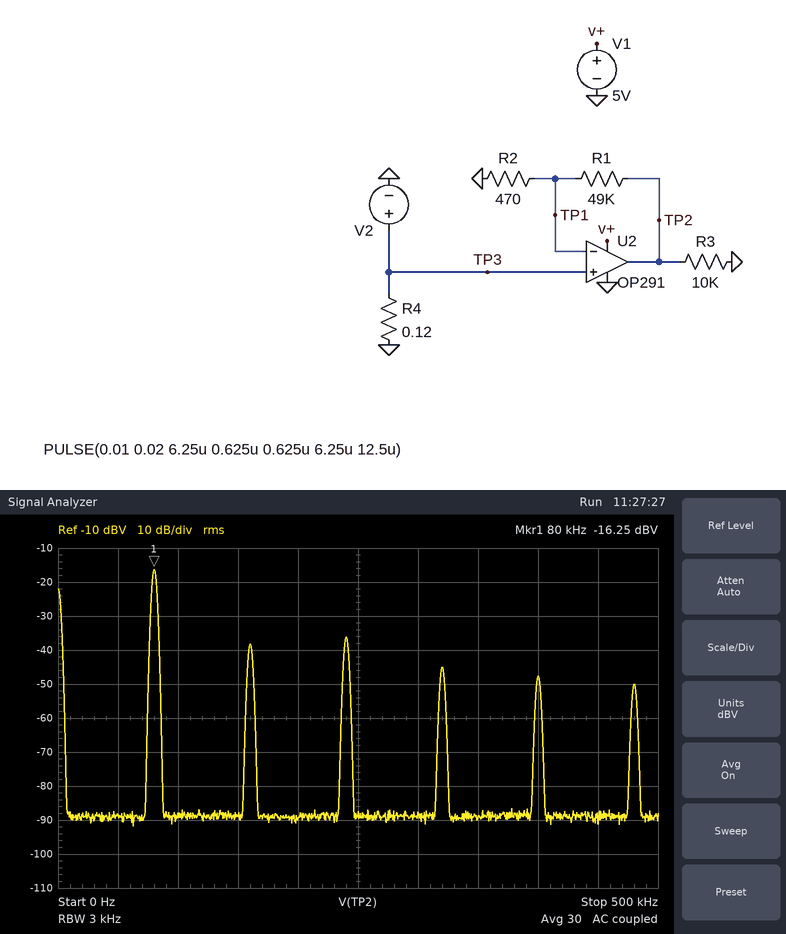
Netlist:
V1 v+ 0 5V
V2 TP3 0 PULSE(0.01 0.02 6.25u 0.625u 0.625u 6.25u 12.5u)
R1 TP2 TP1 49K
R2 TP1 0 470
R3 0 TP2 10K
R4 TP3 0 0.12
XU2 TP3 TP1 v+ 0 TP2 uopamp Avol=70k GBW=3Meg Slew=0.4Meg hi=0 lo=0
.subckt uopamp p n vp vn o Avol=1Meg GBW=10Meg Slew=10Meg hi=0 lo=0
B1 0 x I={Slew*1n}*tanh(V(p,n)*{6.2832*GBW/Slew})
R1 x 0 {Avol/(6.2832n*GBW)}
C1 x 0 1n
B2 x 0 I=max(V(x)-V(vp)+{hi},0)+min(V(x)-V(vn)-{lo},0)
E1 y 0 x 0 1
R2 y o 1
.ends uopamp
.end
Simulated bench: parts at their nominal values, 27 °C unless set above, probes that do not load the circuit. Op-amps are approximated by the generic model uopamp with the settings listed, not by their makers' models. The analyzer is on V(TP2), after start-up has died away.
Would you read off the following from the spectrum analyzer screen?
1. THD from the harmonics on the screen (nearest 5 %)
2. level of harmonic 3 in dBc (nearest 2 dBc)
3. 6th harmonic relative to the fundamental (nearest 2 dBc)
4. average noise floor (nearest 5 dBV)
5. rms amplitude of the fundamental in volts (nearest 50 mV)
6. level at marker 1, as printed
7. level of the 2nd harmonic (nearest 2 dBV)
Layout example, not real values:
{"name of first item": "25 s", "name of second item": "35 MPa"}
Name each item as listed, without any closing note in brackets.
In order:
{"THD from the harmonics on the screen": "15 %", "level of harmonic 3 in dBc": "-20 dBc", "6th harmonic relative to the fundamental": "-34 dBc", "average noise floor": "-90 dBV", "rms amplitude of the fundamental in volts": "150 mV", "level at marker 1, as printed": "-16.25 dBV", "level of the 2nd harmonic": "-38 dBV"}
